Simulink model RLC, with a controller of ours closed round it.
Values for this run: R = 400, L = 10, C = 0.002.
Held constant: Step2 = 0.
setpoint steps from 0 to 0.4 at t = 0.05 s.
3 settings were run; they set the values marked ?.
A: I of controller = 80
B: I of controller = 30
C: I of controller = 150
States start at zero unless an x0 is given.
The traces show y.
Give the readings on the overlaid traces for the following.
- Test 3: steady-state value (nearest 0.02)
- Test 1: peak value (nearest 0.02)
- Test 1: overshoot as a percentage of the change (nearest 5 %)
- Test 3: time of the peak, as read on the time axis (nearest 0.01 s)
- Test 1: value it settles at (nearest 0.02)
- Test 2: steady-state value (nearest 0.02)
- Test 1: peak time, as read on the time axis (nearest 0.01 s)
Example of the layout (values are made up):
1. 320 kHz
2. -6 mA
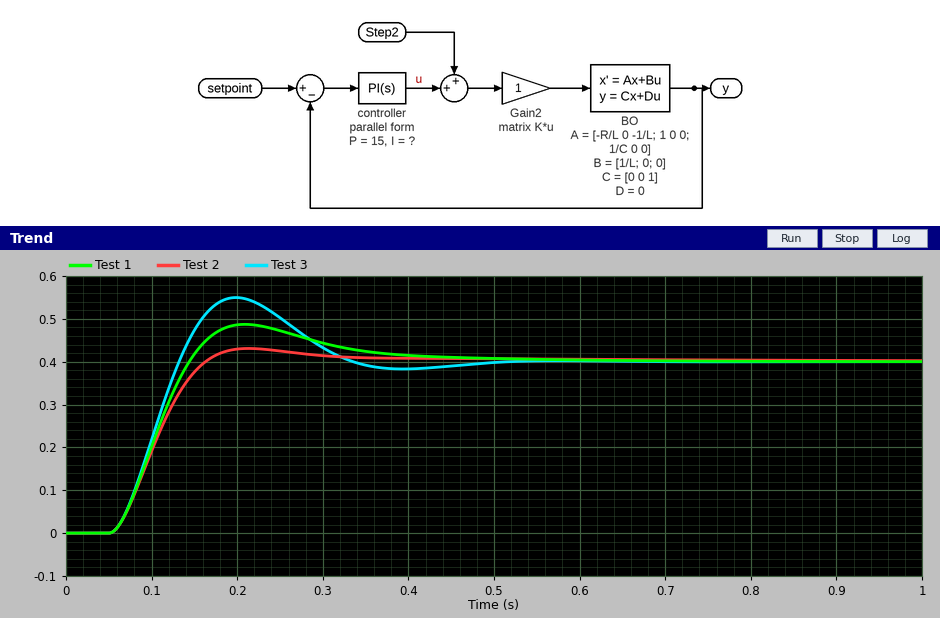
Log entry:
1. 0.40
2. 0.48
3. 20 %
4. 0.20 s
5. 0.40
6. 0.40
7. 0.21 s
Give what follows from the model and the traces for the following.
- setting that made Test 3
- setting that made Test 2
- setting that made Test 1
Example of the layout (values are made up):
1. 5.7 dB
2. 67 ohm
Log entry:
1. C
2. B
3. A
